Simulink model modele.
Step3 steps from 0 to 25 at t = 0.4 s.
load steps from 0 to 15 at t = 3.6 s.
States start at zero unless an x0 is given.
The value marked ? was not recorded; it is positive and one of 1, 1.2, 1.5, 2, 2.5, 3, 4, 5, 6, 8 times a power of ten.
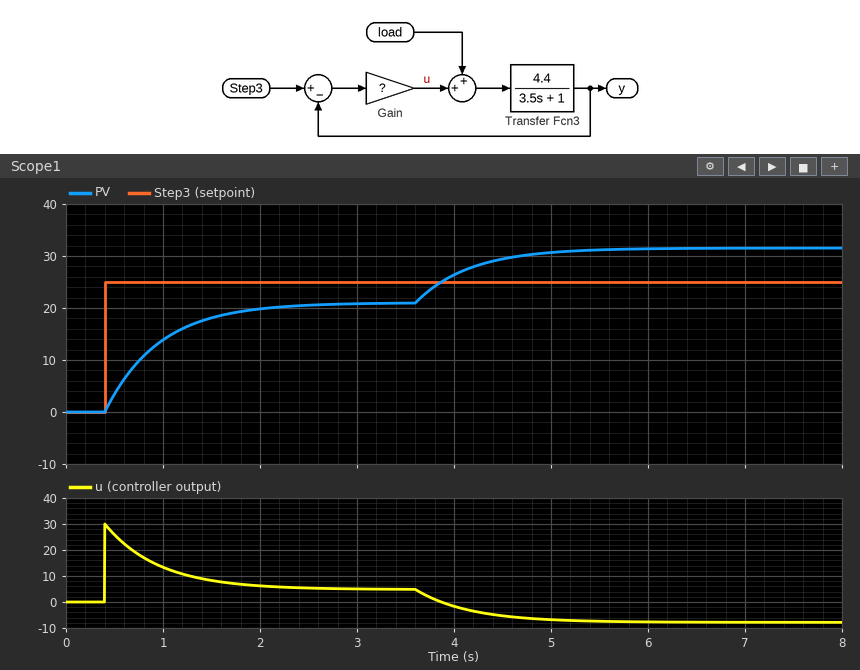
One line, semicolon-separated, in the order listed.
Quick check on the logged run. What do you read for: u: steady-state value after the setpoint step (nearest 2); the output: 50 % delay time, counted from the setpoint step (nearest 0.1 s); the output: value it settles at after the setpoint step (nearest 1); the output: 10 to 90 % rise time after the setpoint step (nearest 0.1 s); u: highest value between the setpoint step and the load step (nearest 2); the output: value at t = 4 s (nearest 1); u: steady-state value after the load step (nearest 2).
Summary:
4; 0.4 s; 21; 1.2 s; 30; 26; -8
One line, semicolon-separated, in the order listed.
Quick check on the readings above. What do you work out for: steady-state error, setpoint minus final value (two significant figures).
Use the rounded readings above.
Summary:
4.0
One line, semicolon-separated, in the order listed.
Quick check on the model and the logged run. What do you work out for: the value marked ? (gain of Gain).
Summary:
1.2
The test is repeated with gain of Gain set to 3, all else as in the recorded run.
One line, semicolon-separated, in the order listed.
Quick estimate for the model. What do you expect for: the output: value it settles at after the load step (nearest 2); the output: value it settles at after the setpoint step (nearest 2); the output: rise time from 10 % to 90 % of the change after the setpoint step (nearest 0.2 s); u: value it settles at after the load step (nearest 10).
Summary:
28; 24; 0.6 s; -10
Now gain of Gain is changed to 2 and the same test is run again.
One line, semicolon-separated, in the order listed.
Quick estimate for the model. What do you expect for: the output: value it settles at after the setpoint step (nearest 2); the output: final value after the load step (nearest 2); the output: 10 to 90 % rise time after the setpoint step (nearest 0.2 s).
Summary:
22; 30; 0.8 s
